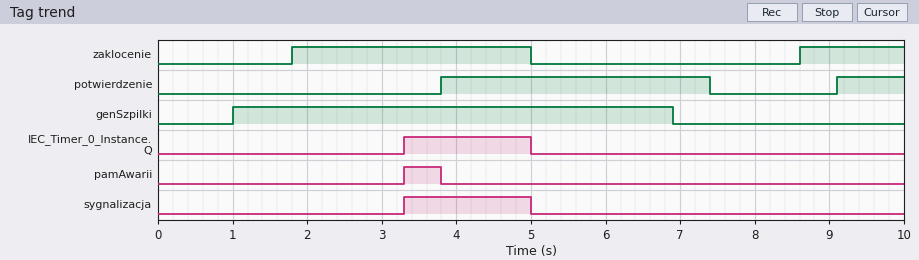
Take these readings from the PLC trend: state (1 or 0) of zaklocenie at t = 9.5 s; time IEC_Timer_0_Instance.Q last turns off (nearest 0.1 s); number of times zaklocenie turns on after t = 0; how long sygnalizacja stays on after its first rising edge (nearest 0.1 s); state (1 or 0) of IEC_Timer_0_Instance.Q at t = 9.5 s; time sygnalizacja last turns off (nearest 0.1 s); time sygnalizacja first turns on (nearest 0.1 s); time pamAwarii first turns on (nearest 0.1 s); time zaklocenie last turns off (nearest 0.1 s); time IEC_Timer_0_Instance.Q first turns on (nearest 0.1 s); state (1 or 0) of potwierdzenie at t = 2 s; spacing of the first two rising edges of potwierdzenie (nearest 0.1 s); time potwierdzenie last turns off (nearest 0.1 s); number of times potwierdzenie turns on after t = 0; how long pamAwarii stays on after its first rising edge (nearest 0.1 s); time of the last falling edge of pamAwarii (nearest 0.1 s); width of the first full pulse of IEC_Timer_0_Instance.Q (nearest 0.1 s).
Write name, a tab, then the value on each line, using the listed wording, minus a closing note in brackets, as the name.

state (1 or 0) of zaklocenie at t = 9.5 s	1
time IEC_Timer_0_Instance.Q last turns off	5.0 s
number of times zaklocenie turns on after t = 0	2
how long sygnalizacja stays on after its first rising edge	1.7 s
state (1 or 0) of IEC_Timer_0_Instance.Q at t = 9.5 s	0
time sygnalizacja last turns off	5.0 s
time sygnalizacja first turns on	3.3 s
time pamAwarii first turns on	3.3 s
time zaklocenie last turns off	5.0 s
time IEC_Timer_0_Instance.Q first turns on	3.3 s
state (1 or 0) of potwierdzenie at t = 2 s	0
spacing of the first two rising edges of potwierdzenie	5.3 s
time potwierdzenie last turns off	7.4 s
number of times potwierdzenie turns on after t = 0	2
how long pamAwarii stays on after its first rising edge	0.5 s
time of the last falling edge of pamAwarii	3.8 s
width of the first full pulse of IEC_Timer_0_Instance.Q	1.7 s
